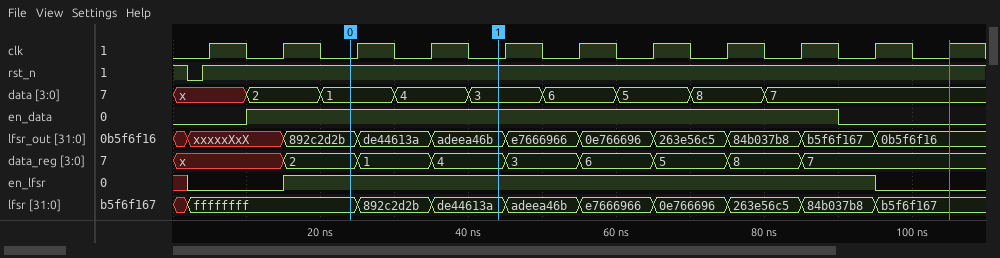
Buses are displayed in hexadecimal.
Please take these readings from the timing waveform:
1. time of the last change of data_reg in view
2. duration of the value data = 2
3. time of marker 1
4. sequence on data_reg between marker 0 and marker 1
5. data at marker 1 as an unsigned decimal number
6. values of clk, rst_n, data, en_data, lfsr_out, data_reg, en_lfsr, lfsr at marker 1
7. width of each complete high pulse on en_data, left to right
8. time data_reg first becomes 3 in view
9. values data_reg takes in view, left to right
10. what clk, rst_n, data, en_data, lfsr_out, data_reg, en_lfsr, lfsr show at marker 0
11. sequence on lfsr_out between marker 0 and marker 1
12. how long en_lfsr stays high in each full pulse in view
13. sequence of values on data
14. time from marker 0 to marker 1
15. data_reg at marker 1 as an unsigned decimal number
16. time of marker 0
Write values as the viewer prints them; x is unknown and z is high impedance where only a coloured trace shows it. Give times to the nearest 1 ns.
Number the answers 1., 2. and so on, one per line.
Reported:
1. 85 ns
2. 10 ns
3. 44 ns
4. 2, 1, 4
5. 3
6. clk=0, rst_n=1, data=3, en_data=1, lfsr_out=adeea46b, data_reg=4, en_lfsr=1, lfsr=de44613a
7. 80 ns
8. 45 ns
9. x, 2, 1, 4, 3, 6, 5, 8, 7
10. clk=0, rst_n=1, data=1, en_data=1, lfsr_out=892c2d2b, data_reg=2, en_lfsr=1, lfsr=ffffffff
11. 892c2d2b, de44613a, adeea46b
12. 80 ns
13. x, 2, 1, 4, 3, 6, 5, 8, 7
14. 20 ns
15. 4
16. 24 ns
